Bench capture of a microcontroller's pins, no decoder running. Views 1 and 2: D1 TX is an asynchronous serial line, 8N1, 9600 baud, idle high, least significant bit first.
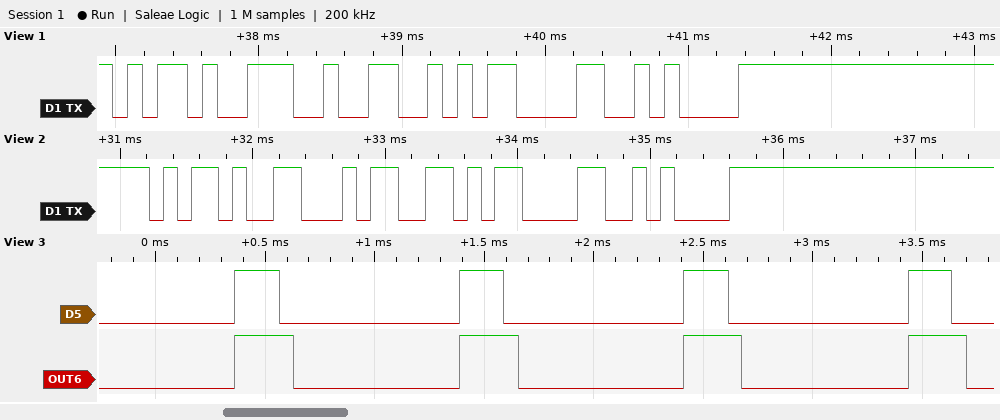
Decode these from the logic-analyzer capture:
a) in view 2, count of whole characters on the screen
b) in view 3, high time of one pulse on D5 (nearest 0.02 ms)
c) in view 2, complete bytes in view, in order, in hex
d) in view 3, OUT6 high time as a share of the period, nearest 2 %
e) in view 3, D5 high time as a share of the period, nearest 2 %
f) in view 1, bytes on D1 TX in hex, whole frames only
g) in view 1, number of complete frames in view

4
0.20 ms
2D 34 0D 0A
26 %
20 %
0x2D 0x32 0x0D 0x0A
4
